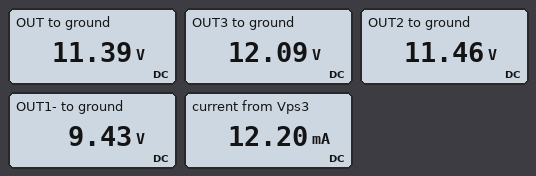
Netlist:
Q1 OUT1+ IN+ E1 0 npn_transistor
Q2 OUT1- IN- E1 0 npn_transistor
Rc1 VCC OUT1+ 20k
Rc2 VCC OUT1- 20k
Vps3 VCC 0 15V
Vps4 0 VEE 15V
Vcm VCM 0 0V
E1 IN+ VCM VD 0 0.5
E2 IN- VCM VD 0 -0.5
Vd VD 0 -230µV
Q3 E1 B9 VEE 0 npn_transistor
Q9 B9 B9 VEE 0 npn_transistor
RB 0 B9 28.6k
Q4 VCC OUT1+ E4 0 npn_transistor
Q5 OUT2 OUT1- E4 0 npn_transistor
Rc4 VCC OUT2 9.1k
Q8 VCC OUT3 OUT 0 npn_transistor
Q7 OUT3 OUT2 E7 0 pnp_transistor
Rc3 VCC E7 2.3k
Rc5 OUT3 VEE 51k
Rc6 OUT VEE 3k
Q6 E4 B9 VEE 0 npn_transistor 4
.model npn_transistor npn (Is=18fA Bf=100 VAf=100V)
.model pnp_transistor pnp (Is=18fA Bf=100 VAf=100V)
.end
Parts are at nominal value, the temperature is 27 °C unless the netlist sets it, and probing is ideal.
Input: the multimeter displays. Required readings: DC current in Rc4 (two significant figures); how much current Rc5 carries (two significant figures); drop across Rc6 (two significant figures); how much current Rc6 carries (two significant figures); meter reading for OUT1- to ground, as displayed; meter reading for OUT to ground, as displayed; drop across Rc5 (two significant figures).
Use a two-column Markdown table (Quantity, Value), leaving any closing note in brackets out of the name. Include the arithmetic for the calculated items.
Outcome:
| Quantity | Value |
|---|---|
| DC current in Rc4 | (15 V - 11.46 V) / 9.1 kΩ = 390 µA |
| how much current Rc5 carries | (12.09 V - (-15 V)) / 51 kΩ = 530 µA |
| drop across Rc6 | 11.39 V - (-15 V) = 26 V |
| how much current Rc6 carries | (11.39 V - (-15 V)) / 3 kΩ = 8.8 mA |
| meter reading for OUT1- to ground, as displayed | 9.43 V |
| meter reading for OUT to ground, as displayed | 11.39 V |
| drop across Rc5 | 12.09 V - (-15 V) = 27 V |
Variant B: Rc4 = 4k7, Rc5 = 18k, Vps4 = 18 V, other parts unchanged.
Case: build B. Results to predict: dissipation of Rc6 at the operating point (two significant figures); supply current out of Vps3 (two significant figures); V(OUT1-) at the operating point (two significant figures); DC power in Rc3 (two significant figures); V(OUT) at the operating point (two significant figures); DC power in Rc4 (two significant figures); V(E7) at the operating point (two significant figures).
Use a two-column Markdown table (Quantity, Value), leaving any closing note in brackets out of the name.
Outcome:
| Quantity | Value |
|---|---|
| dissipation of Rc6 at the operating point | 260 mW |
| supply current out of Vps3 | 14 mA |
| V(OUT1-) at the operating point | 8.1 V |
| DC power in Rc3 | 8.0 mW |
| V(OUT) at the operating point | 9.9 V |
| DC power in Rc4 | 5.2 mW |
| V(E7) at the operating point | 11 V |
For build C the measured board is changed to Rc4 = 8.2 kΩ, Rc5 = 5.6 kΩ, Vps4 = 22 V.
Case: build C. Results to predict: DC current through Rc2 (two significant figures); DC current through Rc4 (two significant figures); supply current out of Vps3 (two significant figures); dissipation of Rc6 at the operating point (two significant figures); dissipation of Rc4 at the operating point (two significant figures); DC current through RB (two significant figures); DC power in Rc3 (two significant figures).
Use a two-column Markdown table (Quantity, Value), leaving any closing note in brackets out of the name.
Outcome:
| Quantity | Value |
|---|---|
| DC current through Rc2 | 440 µA |
| DC current through Rc4 | 1.1 mA |
| supply current out of Vps3 | 15 mA |
| dissipation of Rc6 at the operating point | 130 mW |
| dissipation of Rc4 at the operating point | 11 mW |
| DC current through RB | 750 µA |
| DC power in Rc3 | 33 mW |
